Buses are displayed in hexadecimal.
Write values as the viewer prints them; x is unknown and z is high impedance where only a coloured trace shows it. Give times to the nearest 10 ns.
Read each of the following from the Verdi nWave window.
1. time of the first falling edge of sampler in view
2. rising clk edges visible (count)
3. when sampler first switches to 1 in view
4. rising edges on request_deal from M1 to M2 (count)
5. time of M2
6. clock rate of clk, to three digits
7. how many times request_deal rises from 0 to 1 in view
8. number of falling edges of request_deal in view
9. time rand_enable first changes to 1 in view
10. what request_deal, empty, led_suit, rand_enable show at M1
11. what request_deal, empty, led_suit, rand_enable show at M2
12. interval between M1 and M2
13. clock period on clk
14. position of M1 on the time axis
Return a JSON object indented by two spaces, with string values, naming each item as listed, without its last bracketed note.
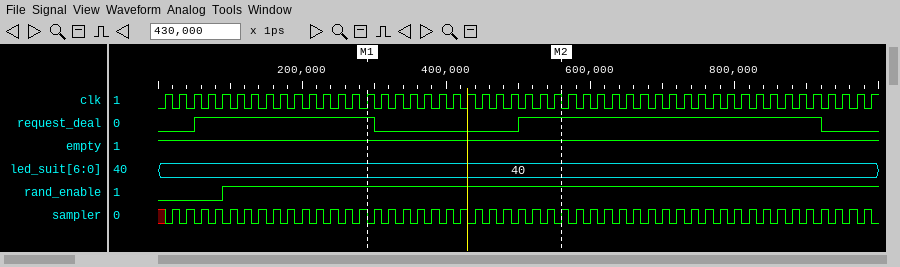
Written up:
{
  "time of the first falling edge of sampler in view": "30 ns",
  "rising clk edges visible": "50",
  "when sampler first switches to 1 in view": "20 ns",
  "rising edges on request_deal from M1 to M2": "1",
  "time of M2": "560 ns",
  "clock rate of clk, to three digits": "50.0 MHz",
  "how many times request_deal rises from 0 to 1 in view": "2",
  "number of falling edges of request_deal in view": "2",
  "time rand_enable first changes to 1 in view": "90 ns",
  "what request_deal, empty, led_suit, rand_enable show at M1": "request_deal=1, empty=1, led_suit=40, rand_enable=1",
  "what request_deal, empty, led_suit, rand_enable show at M2": "request_deal=1, empty=1, led_suit=40, rand_enable=1",
  "interval between M1 and M2": "270 ns",
  "clock period on clk": "20 ns",
  "position of M1 on the time axis": "290 ns"
}
